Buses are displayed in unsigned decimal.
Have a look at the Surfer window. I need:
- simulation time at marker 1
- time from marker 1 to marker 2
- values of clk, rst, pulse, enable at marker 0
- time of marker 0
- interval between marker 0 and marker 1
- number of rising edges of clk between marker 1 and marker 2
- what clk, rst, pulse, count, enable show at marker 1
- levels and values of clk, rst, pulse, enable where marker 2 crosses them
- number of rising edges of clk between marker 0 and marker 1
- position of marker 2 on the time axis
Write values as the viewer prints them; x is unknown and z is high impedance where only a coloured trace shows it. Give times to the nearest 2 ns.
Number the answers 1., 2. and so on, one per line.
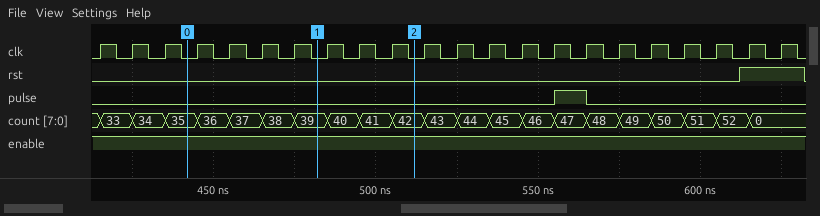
1. 482 ns
2. 30 ns
3. clk=0, rst=0, pulse=0, enable=1
4. 442 ns
5. 40 ns
6. 3
7. clk=0, rst=0, pulse=0, count=39, enable=1
8. clk=0, rst=0, pulse=0, enable=1
9. 4
10. 512 ns
